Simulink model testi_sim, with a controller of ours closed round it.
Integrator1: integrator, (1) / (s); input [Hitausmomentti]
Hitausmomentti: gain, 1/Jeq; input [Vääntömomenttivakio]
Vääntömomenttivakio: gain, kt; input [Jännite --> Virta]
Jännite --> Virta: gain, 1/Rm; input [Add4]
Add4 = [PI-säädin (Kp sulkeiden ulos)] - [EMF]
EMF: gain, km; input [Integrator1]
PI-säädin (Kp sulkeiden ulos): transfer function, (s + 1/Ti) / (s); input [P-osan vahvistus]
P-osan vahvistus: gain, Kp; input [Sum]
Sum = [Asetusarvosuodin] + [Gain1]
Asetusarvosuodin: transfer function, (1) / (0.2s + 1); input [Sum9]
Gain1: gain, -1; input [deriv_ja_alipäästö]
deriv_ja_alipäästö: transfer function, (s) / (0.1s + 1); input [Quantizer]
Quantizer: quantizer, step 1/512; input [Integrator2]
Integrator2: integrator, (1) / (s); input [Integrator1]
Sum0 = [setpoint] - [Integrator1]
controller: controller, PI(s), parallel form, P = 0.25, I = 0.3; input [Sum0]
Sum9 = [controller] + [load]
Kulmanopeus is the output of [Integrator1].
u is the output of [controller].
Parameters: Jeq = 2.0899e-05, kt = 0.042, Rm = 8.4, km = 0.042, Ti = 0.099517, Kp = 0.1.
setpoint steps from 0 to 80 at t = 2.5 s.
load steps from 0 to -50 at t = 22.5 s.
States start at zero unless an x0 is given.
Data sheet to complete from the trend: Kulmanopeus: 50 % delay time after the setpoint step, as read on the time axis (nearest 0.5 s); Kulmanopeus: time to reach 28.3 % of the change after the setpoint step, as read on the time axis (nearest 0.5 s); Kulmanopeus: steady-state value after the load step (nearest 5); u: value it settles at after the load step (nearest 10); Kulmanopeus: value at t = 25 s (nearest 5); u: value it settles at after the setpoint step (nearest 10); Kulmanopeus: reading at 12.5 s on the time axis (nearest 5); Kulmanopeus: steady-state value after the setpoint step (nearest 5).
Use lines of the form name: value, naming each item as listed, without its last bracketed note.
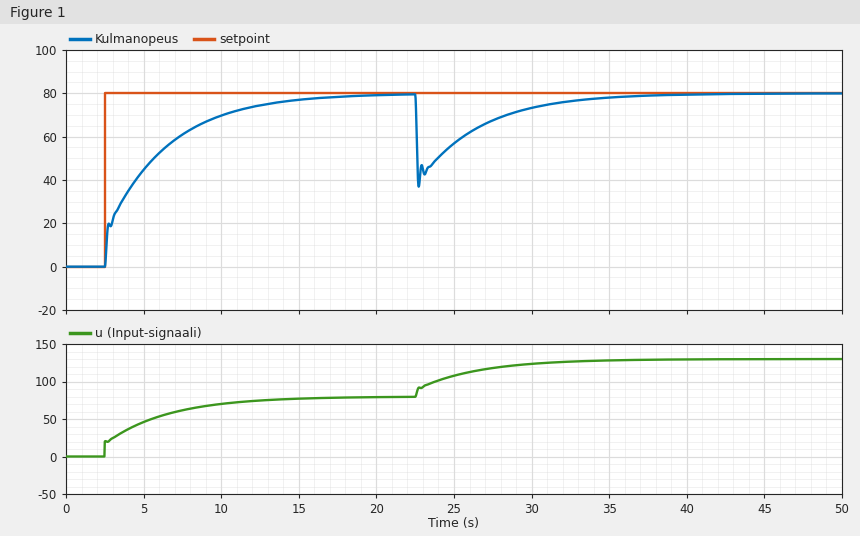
Kulmanopeus: 50 % delay time after the setpoint step, as read on the time axis: 4.5 s
Kulmanopeus: time to reach 28.3 % of the change after the setpoint step, as read on the time axis: 3.0 s
Kulmanopeus: steady-state value after the load step: 80
u: value it settles at after the load step: 130
Kulmanopeus: value at t = 25 s: 55
u: value it settles at after the setpoint step: 80
Kulmanopeus: reading at 12.5 s on the time axis: 75
Kulmanopeus: steady-state value after the setpoint step: 80
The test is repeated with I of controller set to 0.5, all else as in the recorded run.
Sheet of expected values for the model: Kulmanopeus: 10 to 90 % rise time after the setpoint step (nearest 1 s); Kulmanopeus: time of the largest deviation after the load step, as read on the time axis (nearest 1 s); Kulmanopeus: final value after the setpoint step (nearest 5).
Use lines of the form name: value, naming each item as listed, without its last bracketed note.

Kulmanopeus: 10 to 90 % rise time after the setpoint step: 5 s
Kulmanopeus: time of the largest deviation after the load step, as read on the time axis: 23 s
Kulmanopeus: final value after the setpoint step: 80
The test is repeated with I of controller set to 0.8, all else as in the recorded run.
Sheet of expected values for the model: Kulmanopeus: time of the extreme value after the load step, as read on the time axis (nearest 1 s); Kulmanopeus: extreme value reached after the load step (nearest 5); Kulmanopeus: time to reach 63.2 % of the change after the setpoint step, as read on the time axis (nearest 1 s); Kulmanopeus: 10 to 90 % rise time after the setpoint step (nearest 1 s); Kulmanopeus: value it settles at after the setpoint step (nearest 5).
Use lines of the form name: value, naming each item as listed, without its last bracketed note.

Kulmanopeus: time of the extreme value after the load step, as read on the time axis: 23 s
Kulmanopeus: extreme value reached after the load step: 40
Kulmanopeus: time to reach 63.2 % of the change after the setpoint step, as read on the time axis: 4 s
Kulmanopeus: 10 to 90 % rise time after the setpoint step: 3 s
Kulmanopeus: value it settles at after the setpoint step: 80
